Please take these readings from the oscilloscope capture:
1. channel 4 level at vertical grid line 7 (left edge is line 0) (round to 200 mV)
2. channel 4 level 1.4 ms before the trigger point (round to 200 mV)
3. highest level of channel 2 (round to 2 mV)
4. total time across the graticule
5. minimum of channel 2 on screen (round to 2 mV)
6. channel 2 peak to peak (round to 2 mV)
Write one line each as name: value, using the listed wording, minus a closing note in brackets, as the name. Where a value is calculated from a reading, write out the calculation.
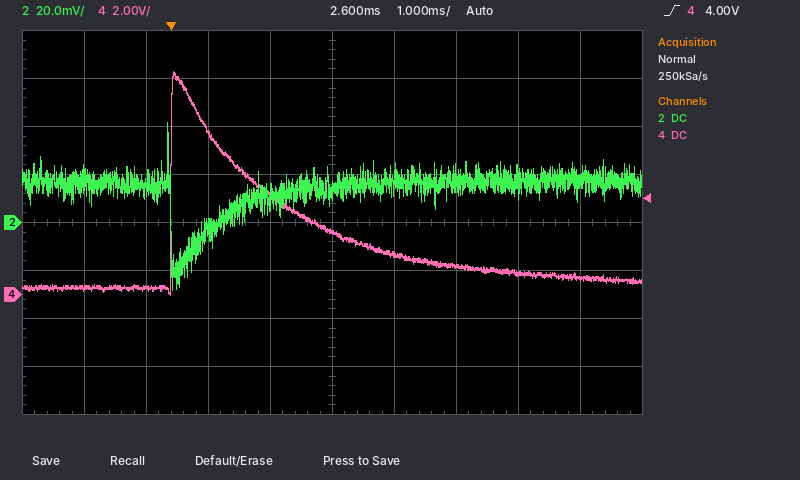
channel 4 level at vertical grid line 7 (left edge is line 0): 1.2 V
channel 4 level 1.4 ms before the trigger point: 200 mV
highest level of channel 2: 42 mV
total time across the graticule: 10 ms
minimum of channel 2 on screen: -28 mV
channel 2 peak to peak: 42 mV − (-28 mV) = 70 mV
